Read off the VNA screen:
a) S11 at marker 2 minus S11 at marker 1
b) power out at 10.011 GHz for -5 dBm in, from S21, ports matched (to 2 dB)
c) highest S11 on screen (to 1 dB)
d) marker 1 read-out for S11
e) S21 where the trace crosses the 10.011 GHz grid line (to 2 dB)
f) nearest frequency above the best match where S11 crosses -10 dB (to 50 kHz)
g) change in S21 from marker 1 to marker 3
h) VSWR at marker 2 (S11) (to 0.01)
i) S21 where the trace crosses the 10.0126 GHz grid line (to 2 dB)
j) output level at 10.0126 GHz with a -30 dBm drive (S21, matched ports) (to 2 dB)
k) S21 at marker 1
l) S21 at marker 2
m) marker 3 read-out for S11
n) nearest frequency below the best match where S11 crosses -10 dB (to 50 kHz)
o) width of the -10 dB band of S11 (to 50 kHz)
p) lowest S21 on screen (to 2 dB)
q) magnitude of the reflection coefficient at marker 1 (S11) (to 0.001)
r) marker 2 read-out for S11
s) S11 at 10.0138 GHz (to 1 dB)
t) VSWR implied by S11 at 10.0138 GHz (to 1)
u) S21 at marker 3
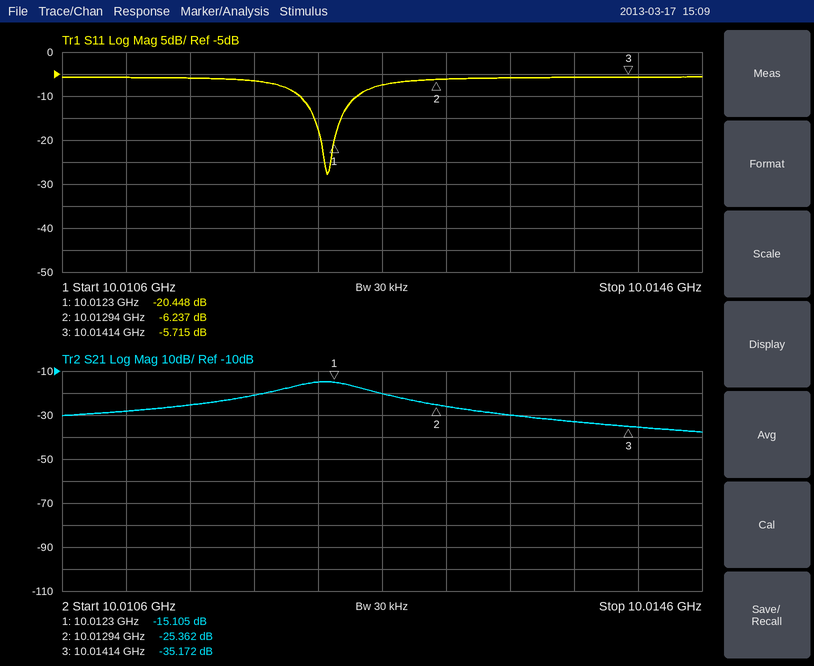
14.211 dB
-34 dBm
-6 dB
-20.448 dB
-28 dB
10.01245 GHz
-20.067 dB
2.90
-20 dB
-50 dBm
-15.105 dB
-25.362 dB
-5.715 dB
10.01210 GHz
350 kHz
-38 dB
0.095
-6.237 dB
-6 dB
3
-35.172 dB
